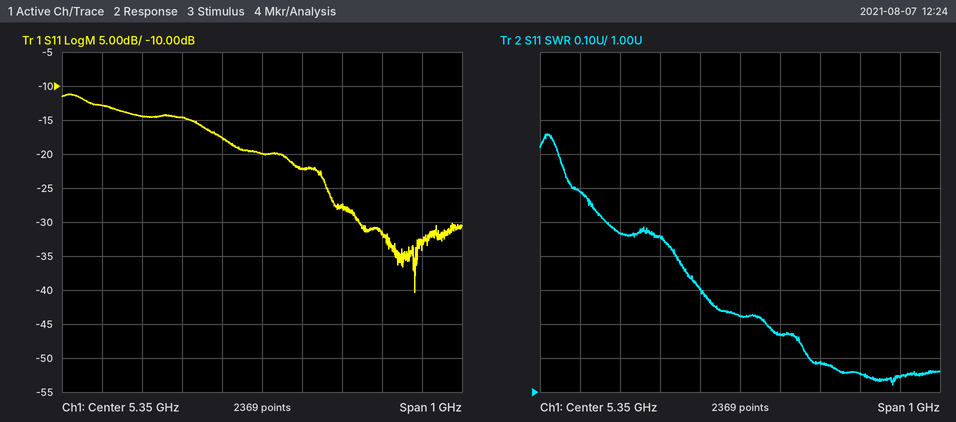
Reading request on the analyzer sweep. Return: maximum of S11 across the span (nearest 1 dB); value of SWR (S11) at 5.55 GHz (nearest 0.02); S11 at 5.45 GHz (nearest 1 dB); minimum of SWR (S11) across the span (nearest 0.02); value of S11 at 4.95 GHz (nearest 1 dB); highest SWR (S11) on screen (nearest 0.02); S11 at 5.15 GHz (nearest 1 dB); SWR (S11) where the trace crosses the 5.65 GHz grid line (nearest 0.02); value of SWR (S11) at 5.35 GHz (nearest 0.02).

-11 dB
1.08
-22 dB
1.02
-13 dB
1.76
-15 dB
1.06
1.22
